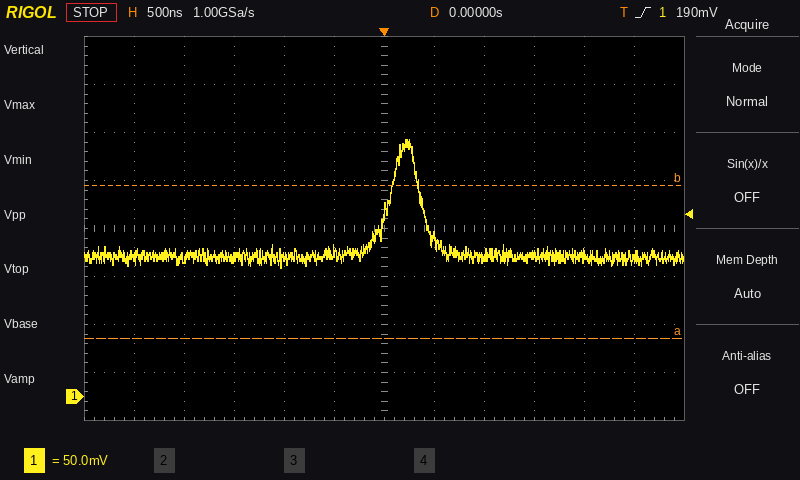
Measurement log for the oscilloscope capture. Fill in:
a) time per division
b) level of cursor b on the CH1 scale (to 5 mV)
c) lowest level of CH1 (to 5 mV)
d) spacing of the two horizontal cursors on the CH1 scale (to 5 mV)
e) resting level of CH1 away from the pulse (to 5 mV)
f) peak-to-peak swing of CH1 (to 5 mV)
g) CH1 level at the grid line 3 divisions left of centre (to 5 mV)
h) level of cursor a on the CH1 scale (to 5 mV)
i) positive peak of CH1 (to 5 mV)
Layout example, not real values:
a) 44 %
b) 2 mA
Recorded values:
a) 500 ns
b) 220 mV
c) 135 mV
d) 160 mV
e) 145 mV
f) 135 mV
g) 145 mV
h) 60 mV
i) 270 mV
